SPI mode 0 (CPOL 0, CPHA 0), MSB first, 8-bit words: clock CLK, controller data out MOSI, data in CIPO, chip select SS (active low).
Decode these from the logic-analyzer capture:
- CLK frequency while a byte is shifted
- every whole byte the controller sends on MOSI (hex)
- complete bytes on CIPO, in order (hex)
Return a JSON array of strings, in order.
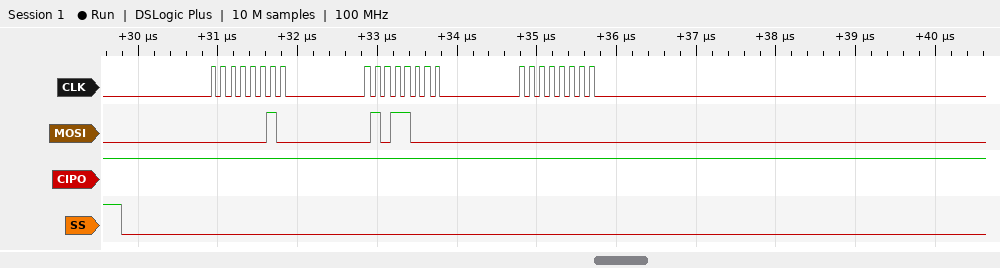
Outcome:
["8 MHz", "02 58 00", "FF FF FF"]
